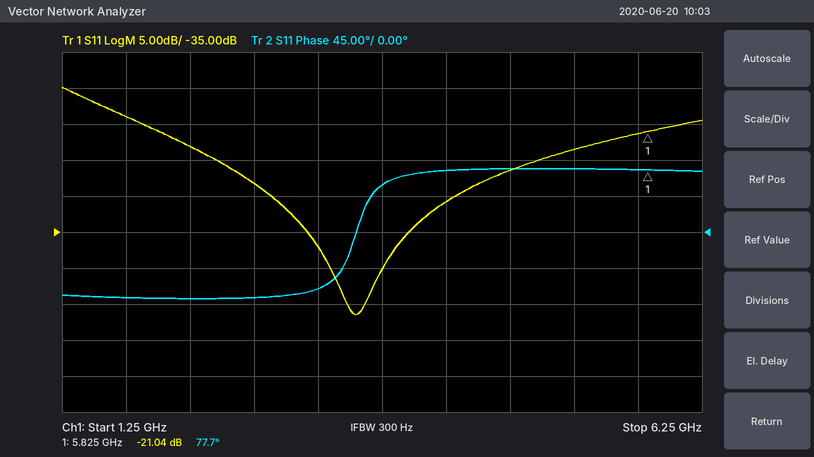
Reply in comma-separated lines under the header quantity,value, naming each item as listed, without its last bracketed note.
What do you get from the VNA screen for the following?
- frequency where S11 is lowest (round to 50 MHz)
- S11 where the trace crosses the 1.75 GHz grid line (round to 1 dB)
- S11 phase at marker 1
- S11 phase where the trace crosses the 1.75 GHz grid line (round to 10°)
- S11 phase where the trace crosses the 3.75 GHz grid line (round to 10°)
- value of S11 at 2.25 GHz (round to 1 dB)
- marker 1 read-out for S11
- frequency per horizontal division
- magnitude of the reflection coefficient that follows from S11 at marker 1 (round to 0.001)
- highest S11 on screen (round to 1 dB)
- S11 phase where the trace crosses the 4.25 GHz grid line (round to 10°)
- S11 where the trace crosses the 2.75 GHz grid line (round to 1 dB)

quantity,value
frequency where S11 is lowest,3.55 GHz
S11 where the trace crosses the 1.75 GHz grid line,-19 dB
S11 phase at marker 1,77.7°
S11 phase where the trace crosses the 1.75 GHz grid line,-80°
S11 phase where the trace crosses the 3.75 GHz grid line,60°
value of S11 at 2.25 GHz,-23 dB
marker 1 read-out for S11,-21.04 dB
frequency per horizontal division,500 MHz
magnitude of the reflection coefficient that follows from S11 at marker 1,0.089
highest S11 on screen,-15 dB
S11 phase where the trace crosses the 4.25 GHz grid line,80°
S11 where the trace crosses the 2.75 GHz grid line,-28 dB
